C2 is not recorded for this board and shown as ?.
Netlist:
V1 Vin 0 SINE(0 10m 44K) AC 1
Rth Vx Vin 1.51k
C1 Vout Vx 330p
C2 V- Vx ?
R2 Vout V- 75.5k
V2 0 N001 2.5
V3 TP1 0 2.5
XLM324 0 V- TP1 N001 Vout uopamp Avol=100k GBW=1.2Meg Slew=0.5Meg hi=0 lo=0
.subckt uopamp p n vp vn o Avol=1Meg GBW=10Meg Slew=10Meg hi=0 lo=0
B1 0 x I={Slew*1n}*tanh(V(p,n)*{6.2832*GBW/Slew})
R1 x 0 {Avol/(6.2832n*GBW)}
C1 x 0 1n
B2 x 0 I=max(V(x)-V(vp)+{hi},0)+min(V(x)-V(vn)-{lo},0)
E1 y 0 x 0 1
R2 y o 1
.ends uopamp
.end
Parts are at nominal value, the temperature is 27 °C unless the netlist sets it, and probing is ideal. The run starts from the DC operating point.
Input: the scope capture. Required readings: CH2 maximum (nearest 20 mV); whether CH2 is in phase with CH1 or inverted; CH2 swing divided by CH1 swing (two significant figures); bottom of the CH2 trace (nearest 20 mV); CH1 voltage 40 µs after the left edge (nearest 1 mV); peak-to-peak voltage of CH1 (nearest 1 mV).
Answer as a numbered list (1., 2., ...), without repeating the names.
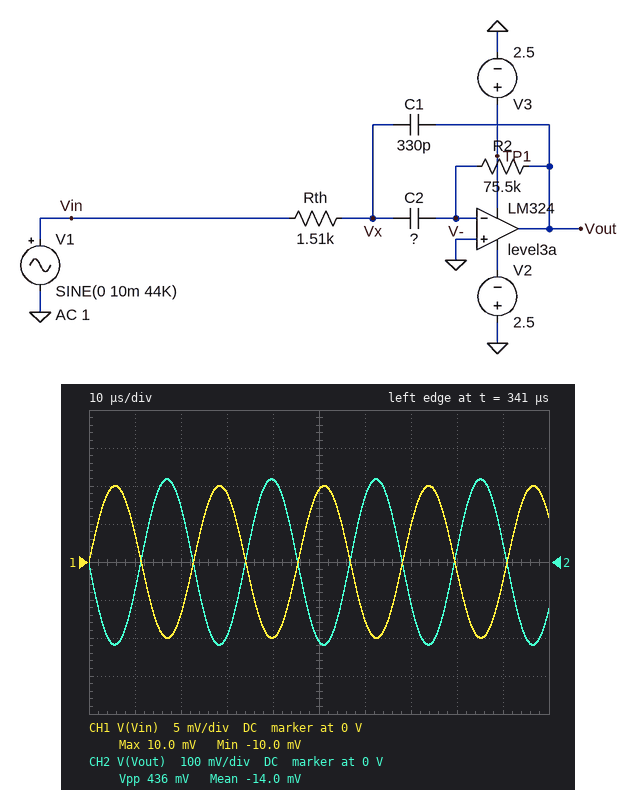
1. 220 mV
2. inverted
3. 22
4. -220 mV
5. -10 mV
6. 20 mV
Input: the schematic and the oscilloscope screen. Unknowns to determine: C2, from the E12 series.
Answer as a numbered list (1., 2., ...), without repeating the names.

1. 270 pF
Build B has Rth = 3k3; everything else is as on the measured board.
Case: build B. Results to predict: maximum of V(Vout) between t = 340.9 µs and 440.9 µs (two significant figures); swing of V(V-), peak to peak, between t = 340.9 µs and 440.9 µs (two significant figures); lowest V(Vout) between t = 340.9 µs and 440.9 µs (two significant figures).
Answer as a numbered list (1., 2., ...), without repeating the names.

1. 53 mV
2. 3.9 mV
3. -53 mV
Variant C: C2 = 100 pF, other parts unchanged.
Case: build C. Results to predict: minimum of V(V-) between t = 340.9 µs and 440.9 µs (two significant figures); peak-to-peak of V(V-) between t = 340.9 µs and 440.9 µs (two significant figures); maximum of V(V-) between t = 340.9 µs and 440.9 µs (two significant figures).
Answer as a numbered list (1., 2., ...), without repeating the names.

1. -1.2 mV
2. 2.3 mV
3. 1.2 mV
